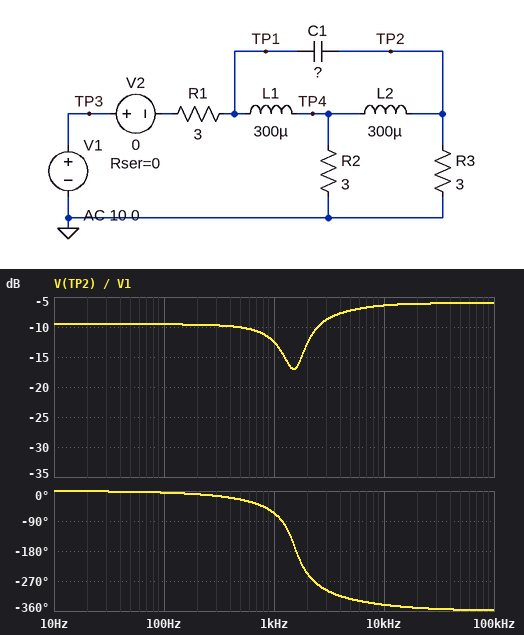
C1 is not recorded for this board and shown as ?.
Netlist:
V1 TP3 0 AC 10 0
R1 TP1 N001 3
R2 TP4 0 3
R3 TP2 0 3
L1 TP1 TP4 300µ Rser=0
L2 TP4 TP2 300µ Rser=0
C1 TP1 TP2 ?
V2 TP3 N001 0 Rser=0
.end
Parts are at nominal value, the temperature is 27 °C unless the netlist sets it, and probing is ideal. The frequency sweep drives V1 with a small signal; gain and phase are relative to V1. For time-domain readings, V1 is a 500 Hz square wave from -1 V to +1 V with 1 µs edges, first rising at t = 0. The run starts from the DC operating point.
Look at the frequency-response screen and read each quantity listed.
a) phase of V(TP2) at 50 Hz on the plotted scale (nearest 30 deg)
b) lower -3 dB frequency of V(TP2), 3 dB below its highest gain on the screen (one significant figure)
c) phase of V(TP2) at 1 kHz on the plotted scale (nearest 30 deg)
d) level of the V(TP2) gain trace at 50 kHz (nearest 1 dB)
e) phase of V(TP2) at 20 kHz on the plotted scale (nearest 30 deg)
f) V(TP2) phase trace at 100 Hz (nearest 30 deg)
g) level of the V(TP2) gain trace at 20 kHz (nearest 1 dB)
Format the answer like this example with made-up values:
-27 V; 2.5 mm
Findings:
0 deg; 3 kHz; -60 deg; -6 dB; -360 deg; 0 deg; -6 dB
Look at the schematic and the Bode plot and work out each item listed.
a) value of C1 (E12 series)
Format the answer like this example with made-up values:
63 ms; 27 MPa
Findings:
15 µF
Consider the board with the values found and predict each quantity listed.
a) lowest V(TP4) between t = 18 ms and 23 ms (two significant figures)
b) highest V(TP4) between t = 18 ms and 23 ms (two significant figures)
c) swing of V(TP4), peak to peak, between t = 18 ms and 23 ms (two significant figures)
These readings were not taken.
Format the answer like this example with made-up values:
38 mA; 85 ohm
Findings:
-330 mV; 330 mV; 670 mV
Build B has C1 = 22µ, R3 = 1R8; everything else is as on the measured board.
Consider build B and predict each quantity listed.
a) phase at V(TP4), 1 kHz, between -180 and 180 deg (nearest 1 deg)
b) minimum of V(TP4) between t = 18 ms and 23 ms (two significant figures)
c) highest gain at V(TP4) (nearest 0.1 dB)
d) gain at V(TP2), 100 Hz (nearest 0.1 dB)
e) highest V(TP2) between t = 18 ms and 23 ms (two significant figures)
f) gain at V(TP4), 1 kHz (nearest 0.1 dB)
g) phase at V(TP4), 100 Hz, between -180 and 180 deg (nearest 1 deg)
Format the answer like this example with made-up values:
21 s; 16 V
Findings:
-6 deg; -360 mV; -9.3 dB; -11.3 dB; 480 mV; -9.7 dB; 0 deg
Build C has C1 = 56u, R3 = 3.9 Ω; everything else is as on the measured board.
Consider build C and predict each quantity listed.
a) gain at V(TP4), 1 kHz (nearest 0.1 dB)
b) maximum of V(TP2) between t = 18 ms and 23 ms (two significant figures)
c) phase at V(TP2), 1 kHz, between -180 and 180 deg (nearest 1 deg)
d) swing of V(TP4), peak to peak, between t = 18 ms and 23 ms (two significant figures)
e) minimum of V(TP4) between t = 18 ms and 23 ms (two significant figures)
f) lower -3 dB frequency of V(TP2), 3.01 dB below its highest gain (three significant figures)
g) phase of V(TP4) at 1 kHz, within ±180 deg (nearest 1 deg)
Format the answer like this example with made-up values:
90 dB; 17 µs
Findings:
-9.8 dB; 670 mV; 100 deg; 750 mV; -370 mV; 1.67 kHz; -8 deg
